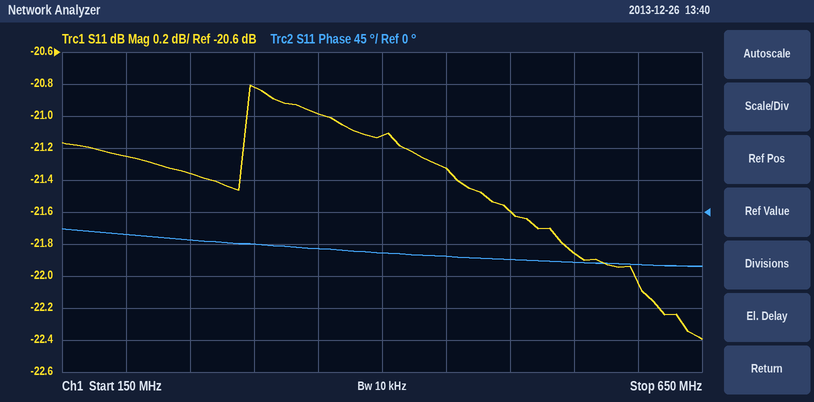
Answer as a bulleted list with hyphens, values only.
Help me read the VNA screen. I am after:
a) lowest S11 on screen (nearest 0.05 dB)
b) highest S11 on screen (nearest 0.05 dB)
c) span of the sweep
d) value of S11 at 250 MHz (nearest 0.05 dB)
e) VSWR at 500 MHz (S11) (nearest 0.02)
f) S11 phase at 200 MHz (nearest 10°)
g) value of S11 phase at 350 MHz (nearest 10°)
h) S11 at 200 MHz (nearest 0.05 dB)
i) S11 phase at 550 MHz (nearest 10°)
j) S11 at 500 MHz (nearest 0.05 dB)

- -22.40 dB
- -20.80 dB
- 500 MHz
- -21.35 dB
- 1.18
- -30°
- -50°
- -21.25 dB
- -70°
- -21.60 dB
